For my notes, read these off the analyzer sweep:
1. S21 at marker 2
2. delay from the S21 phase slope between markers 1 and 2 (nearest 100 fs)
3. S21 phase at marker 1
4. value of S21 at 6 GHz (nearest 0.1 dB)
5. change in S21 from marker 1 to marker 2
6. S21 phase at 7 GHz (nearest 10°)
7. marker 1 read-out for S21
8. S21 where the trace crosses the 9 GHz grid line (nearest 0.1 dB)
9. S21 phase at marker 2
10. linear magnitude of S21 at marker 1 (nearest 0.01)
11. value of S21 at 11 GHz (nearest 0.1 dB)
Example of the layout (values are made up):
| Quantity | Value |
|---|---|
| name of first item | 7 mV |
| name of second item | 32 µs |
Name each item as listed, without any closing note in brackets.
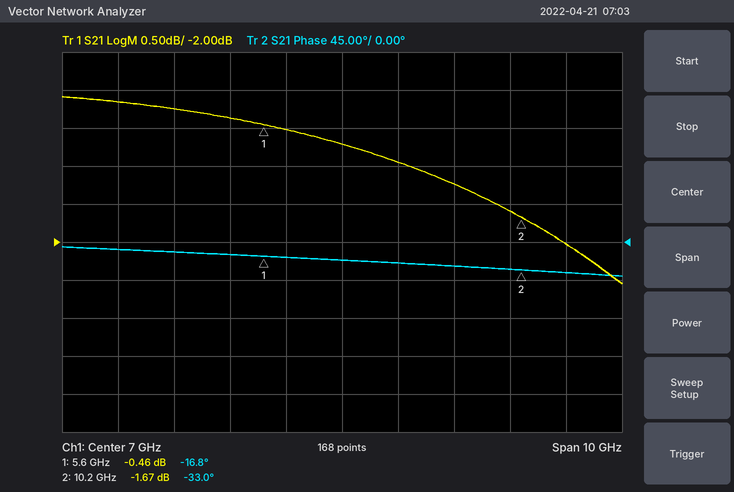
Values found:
| Quantity | Value |
|---|---|
| S21 at marker 2 | -1.67 dB |
| delay from the S21 phase slope between markers 1 and 2 | 9.8 ps |
| S21 phase at marker 1 | -16.8° |
| value of S21 at 6 GHz | -0.5 dB |
| change in S21 from marker 1 to marker 2 | -1.21 dB |
| S21 phase at 7 GHz | -20° |
| marker 1 read-out for S21 | -0.46 dB |
| S21 where the trace crosses the 9 GHz grid line | -1.2 dB |
| S21 phase at marker 2 | -33.0° |
| linear magnitude of S21 at marker 1 | 0.95 |
| value of S21 at 11 GHz | -2.0 dB |
